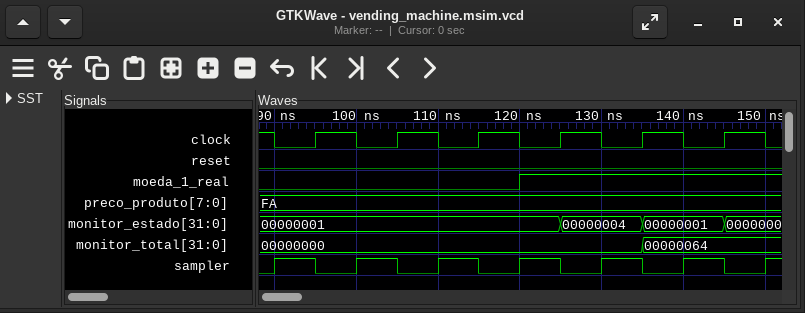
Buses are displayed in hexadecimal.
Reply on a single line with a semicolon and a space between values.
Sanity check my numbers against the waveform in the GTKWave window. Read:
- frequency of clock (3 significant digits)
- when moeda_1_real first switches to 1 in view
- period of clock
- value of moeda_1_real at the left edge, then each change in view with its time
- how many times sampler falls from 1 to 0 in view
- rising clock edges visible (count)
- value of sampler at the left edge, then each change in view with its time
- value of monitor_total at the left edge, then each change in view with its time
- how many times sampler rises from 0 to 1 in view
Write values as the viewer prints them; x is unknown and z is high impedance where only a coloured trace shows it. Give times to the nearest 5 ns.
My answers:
100 MHz; 120 ns; 10 ns; 0, 1 at 120 ns; 6; 6; 0, 1 at 90 ns, 0 at 95 ns, 1 at 100 ns, 0 at 105 ns, 1 at 110 ns, 0 at 115 ns, 1 at 120 ns, 0 at 125 ns, 1 at 130 ns, 0 at 135 ns, 1 at 140 ns, 0 at 145 ns, 1 at 150 ns; 00000000, 00000064 at 135 ns; 7
